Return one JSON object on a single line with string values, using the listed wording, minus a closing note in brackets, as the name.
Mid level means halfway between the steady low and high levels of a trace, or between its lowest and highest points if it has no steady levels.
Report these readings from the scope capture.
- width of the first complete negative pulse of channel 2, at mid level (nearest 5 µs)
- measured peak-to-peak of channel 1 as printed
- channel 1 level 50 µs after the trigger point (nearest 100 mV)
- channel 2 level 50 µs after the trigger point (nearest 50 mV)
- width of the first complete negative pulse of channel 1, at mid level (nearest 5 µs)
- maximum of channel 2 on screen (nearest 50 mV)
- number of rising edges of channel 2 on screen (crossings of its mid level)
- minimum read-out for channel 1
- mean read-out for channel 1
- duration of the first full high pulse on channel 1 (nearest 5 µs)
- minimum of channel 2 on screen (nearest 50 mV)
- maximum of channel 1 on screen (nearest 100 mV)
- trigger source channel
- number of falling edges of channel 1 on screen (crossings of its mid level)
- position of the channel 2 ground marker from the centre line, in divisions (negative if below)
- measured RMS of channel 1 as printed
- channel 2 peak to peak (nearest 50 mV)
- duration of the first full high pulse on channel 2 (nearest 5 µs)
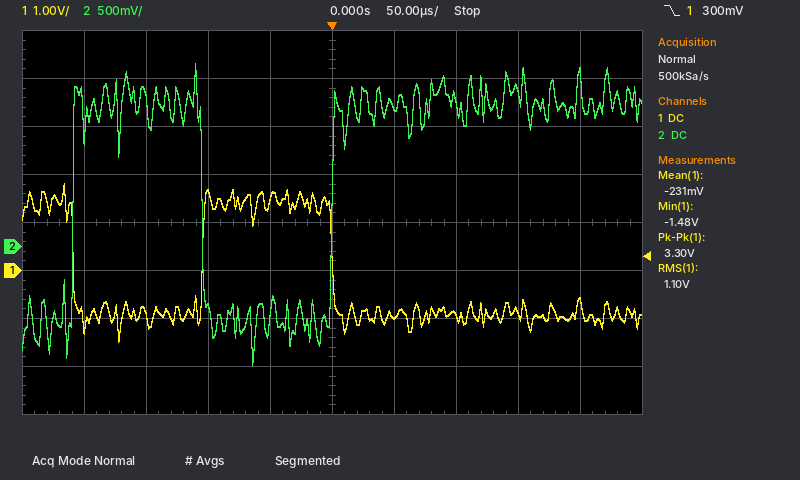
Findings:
{"width of the first complete negative pulse of channel 2, at mid level": "105 µs", "measured peak-to-peak of channel 1 as printed": "3.30 V", "channel 1 level 50 µs after the trigger point": "-1.0 V", "channel 2 level 50 µs after the trigger point": "1.45 V", "width of the first complete negative pulse of channel 1, at mid level": "105 µs", "maximum of channel 2 on screen": "1.90 V", "number of rising edges of channel 2 on screen": "2", "minimum read-out for channel 1": "-1.48 V", "mean read-out for channel 1": "-231 mV", "duration of the first full high pulse on channel 1": "105 µs", "minimum of channel 2 on screen": "-1.25 V", "maximum of channel 1 on screen": "1.8 V", "trigger source channel": "channel 1", "number of falling edges of channel 1 on screen": "2", "position of the channel 2 ground marker from the centre line, in divisions": "-0.5 div", "measured RMS of channel 1 as printed": "1.10 V", "channel 2 peak to peak": "3.15 V", "duration of the first full high pulse on channel 2": "105 µs"}
